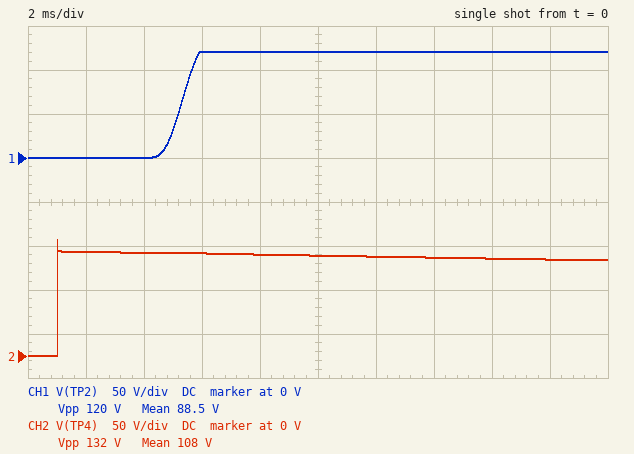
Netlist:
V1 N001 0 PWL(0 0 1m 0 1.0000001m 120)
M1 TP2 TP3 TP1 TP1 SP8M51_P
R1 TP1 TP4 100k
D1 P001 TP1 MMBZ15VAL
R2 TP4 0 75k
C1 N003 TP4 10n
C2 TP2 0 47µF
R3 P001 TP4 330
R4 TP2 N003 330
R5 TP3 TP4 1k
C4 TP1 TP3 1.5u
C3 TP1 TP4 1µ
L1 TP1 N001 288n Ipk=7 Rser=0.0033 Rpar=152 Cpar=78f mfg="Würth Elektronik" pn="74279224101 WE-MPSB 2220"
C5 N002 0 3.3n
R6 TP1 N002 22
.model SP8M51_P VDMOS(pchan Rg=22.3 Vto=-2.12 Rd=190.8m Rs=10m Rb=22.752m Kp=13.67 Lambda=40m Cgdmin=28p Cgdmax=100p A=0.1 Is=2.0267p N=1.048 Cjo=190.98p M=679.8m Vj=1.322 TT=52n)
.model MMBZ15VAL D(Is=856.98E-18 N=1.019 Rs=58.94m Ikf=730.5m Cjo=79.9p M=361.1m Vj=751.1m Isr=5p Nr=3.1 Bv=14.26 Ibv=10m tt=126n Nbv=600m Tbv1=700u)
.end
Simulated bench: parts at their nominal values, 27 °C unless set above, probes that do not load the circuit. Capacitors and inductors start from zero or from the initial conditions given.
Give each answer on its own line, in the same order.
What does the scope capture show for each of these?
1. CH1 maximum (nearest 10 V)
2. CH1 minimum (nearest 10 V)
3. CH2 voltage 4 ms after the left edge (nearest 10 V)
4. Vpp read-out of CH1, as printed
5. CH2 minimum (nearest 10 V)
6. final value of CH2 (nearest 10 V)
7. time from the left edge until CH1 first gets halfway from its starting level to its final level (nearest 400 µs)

120 V
0 V
120 V
120 V
0 V
110 V
5.2 ms
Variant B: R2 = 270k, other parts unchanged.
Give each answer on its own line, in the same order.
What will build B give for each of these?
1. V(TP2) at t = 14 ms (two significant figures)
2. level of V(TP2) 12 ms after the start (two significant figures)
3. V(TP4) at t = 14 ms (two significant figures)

61 V
6.8 V
120 V
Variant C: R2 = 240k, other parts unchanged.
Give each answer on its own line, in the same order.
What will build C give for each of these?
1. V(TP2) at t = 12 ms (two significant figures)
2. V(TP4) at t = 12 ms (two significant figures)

37 V
120 V
